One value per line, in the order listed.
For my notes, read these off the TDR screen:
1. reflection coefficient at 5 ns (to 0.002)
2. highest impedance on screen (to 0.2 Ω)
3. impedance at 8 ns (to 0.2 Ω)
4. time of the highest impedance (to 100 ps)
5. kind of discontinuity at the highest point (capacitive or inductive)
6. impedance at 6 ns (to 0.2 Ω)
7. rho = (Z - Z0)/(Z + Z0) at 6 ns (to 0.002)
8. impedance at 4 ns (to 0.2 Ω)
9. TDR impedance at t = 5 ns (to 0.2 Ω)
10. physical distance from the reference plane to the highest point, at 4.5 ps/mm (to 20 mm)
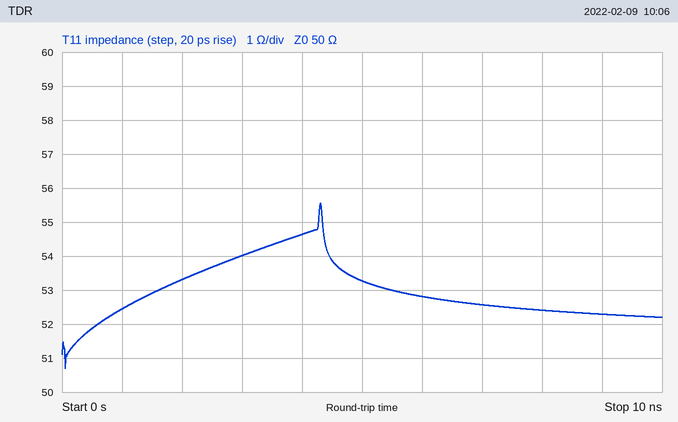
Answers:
+0.032
55.6 Ω
52.4 Ω
4.3 ns
inductive
52.8 Ω
+0.028
54.6 Ω
53.2 Ω
480 mm
